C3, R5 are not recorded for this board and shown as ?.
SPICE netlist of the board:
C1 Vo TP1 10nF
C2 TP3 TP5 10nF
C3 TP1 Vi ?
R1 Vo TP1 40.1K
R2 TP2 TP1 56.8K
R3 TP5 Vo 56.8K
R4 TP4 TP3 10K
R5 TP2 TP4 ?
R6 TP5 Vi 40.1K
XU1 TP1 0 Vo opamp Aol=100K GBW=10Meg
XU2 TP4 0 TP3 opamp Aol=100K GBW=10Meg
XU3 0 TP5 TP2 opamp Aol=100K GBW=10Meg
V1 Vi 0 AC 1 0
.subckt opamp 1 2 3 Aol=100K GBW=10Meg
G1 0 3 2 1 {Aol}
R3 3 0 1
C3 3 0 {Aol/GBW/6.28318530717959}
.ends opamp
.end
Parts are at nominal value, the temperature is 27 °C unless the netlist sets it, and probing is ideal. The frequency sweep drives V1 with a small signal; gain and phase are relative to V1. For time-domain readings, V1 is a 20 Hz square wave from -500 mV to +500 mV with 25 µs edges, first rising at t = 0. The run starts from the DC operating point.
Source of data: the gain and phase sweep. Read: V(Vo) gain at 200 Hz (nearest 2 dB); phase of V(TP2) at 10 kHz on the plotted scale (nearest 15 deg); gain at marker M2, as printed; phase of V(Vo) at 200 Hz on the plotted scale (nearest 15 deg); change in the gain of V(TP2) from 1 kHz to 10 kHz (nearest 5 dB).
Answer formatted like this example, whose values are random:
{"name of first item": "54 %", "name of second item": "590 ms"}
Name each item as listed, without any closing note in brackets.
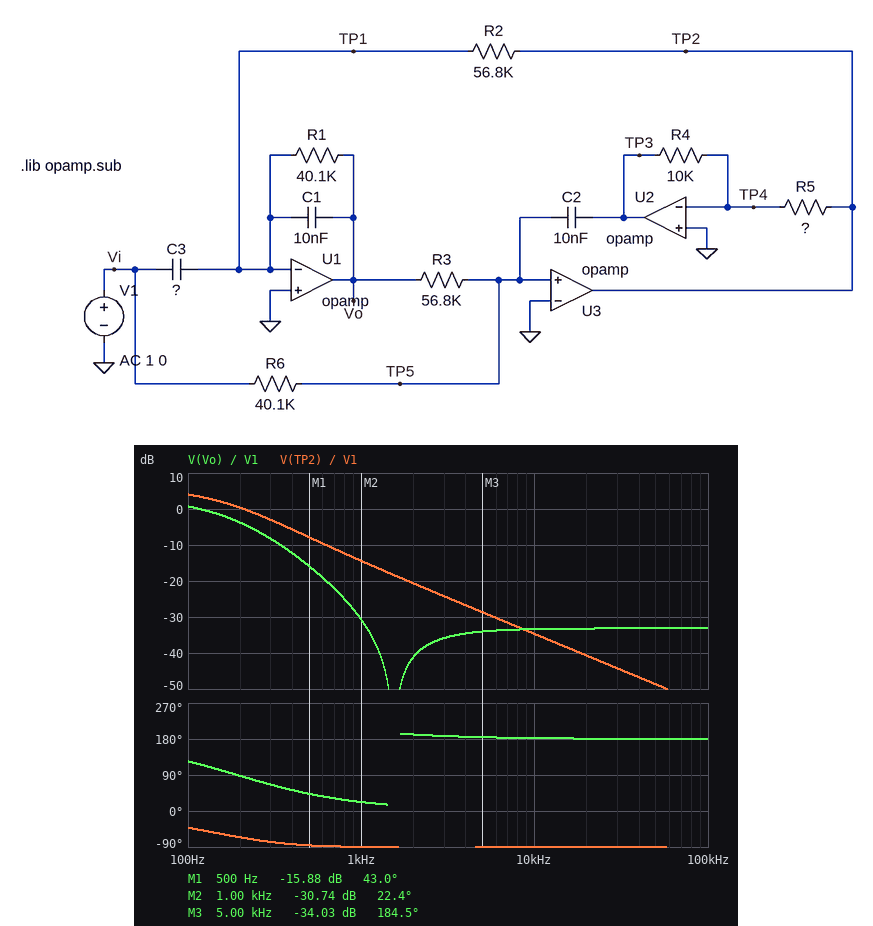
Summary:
{"V(Vo) gain at 200 Hz": "-4 dB", "phase of V(TP2) at 10 kHz on the plotted scale": "-90 deg", "gain at marker M2, as printed": "-30.74 dB", "phase of V(Vo) at 200 Hz on the plotted scale": "90 deg", "change in the gain of V(TP2) from 1 kHz to 10 kHz": "-20 dB"}
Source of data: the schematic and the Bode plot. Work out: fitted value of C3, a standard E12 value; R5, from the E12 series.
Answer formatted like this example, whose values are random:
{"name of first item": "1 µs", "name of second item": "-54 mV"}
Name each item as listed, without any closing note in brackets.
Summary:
{"fitted value of C3, a standard E12 value": "220 pF", "R5, from the E12 series": "4.7 kΩ"}
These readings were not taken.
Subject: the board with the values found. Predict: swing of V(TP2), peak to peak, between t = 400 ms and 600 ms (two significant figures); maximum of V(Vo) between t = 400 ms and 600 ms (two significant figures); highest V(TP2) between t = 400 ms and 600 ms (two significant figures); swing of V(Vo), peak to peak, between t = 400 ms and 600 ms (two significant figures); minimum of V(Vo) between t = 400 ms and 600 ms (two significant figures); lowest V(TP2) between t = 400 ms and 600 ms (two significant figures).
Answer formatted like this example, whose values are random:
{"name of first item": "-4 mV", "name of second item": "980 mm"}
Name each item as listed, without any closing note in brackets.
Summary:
{"swing of V(TP2), peak to peak, between t = 400 ms and 600 ms": "2.0 V", "maximum of V(Vo) between t = 400 ms and 600 ms": "710 mV", "highest V(TP2) between t = 400 ms and 600 ms": "1.0 V", "swing of V(Vo), peak to peak, between t = 400 ms and 600 ms": "1.4 V", "minimum of V(Vo) between t = 400 ms and 600 ms": "-710 mV", "lowest V(TP2) between t = 400 ms and 600 ms": "-1.0 V"}
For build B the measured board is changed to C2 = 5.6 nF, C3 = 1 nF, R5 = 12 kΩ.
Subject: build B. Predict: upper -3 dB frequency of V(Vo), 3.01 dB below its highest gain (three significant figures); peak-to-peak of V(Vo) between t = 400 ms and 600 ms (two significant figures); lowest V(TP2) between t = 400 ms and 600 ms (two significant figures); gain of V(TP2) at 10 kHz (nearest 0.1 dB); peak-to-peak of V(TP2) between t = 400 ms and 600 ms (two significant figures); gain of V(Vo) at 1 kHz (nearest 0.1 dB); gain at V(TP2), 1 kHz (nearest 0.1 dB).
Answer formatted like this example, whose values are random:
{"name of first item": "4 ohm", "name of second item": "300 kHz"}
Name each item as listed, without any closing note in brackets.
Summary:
{"upper -3 dB frequency of V(Vo), 3.01 dB below its highest gain": "464 Hz", "peak-to-peak of V(Vo) between t = 400 ms and 600 ms": "1.9 V", "lowest V(TP2) between t = 400 ms and 600 ms": "-1.6 V", "gain of V(TP2) at 10 kHz": "-22.0 dB", "peak-to-peak of V(TP2) between t = 400 ms and 600 ms": "3.3 V", "gain of V(Vo) at 1 kHz": "-16.5 dB", "gain at V(TP2), 1 kHz": "-0.6 dB"}
